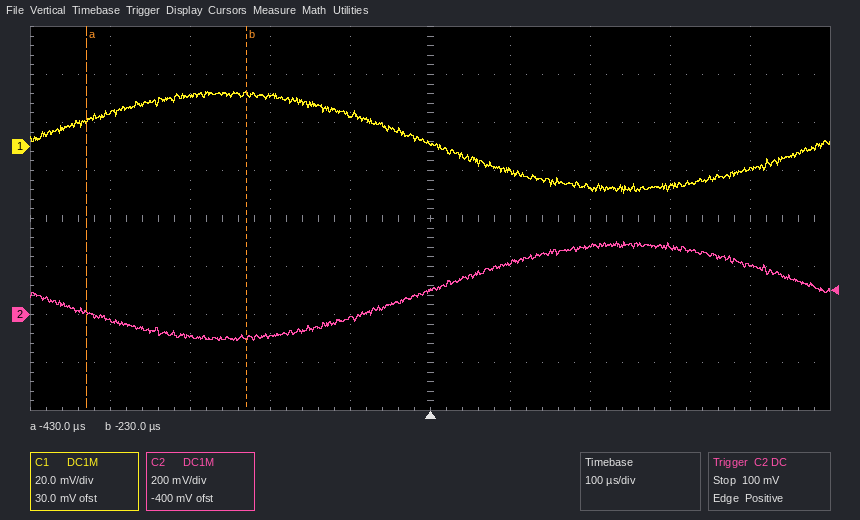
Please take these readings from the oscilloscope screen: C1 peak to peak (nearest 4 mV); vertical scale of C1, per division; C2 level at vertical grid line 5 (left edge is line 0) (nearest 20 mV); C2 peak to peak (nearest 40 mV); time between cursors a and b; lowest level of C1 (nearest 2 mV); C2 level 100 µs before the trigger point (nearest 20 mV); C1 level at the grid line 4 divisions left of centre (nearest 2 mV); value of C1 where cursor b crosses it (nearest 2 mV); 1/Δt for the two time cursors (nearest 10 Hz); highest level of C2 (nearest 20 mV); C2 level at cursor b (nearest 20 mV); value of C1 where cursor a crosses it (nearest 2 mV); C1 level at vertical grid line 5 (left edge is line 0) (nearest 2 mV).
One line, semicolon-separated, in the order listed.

44 mV; 20 mV; 100 mV; 400 mV; 200 µs; -20 mV; -20 mV; 14 mV; 22 mV; 5.00 kHz; 300 mV; -100 mV; 10 mV; 2 mV
